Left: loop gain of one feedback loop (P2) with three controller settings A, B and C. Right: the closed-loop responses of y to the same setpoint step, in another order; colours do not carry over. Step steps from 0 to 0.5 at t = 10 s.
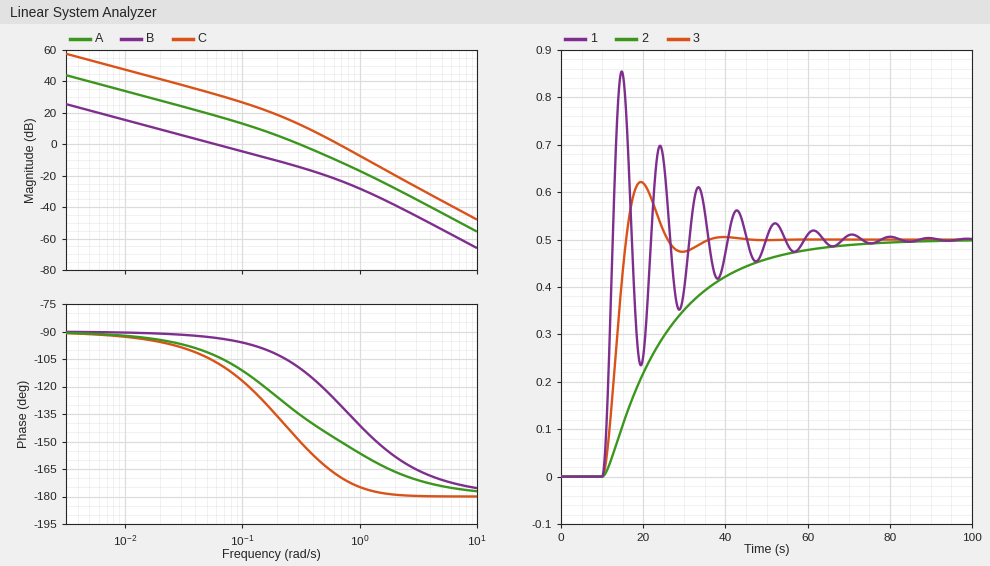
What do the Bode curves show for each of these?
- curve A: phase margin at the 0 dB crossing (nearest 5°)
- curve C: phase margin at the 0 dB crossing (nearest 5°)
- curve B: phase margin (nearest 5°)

45°
10°
85°
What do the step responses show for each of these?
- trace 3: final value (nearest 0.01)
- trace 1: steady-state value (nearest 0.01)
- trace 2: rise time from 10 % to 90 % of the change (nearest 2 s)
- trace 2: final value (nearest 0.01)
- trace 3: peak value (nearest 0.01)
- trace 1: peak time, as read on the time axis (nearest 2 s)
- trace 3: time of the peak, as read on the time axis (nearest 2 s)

0.50
0.50
34 s
0.50
0.62
14 s
20 s
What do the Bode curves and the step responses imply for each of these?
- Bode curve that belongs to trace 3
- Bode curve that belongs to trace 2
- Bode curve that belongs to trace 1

A
B
C
